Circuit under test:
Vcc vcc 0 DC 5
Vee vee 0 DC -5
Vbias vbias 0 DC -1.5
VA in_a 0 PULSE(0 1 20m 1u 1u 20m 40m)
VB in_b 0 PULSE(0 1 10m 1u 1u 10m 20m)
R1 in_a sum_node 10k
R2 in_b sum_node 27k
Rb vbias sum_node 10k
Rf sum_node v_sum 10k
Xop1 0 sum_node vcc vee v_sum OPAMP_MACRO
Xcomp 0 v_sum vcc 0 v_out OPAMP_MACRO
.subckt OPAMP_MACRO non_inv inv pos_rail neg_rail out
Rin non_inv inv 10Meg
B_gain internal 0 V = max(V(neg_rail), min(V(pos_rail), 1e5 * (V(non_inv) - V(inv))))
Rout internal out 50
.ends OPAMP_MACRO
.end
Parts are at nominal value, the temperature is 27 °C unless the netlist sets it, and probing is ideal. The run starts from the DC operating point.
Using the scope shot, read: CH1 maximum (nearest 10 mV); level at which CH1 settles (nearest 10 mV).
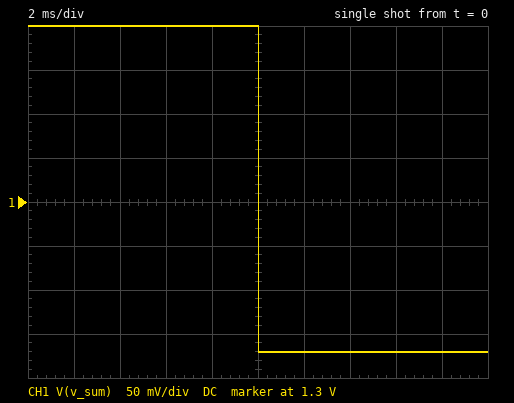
1.50 V
1.13 V
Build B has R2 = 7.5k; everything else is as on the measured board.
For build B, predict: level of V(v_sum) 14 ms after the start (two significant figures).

170 mV
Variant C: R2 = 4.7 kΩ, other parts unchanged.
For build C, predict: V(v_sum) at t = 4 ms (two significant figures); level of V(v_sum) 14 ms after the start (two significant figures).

1.5 V
-630 mV
